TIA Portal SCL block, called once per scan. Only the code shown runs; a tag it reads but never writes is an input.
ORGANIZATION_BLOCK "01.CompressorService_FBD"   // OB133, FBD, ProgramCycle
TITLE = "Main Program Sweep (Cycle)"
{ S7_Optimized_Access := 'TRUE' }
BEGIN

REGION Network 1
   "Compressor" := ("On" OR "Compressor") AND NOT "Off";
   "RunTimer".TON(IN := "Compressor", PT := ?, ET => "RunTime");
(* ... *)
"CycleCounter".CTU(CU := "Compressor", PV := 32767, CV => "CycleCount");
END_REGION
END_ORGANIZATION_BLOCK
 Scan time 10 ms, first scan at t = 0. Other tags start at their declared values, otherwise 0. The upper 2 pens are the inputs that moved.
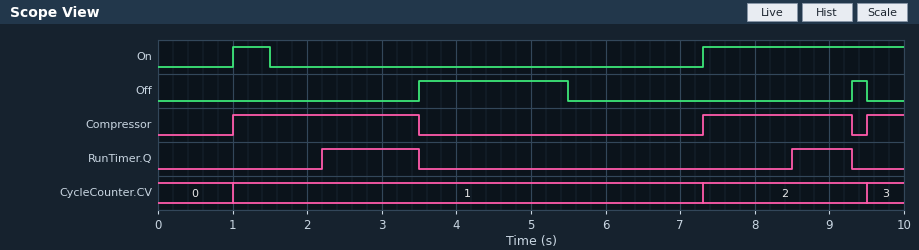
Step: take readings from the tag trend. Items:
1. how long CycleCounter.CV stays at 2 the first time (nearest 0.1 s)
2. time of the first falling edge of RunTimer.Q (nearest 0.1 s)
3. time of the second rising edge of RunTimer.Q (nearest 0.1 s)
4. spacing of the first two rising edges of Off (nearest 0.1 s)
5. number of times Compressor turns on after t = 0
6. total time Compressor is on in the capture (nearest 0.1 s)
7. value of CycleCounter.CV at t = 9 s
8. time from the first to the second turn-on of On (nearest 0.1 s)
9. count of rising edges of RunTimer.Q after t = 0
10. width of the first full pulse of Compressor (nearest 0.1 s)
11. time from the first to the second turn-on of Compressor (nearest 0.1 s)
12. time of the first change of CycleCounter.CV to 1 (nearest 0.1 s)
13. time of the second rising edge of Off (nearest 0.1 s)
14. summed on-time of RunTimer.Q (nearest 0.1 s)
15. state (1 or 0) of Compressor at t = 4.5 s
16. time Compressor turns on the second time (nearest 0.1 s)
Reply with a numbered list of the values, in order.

1. 2.2 s
2. 3.5 s
3. 8.5 s
4. 5.8 s
5. 3
6. 5.0 s
7. 2
8. 6.3 s
9. 2
10. 2.5 s
11. 6.3 s
12. 1.0 s
13. 9.3 s
14. 2.1 s
15. 0
16. 7.3 s
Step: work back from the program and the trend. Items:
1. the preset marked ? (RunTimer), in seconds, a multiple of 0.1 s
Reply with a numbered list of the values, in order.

1. 1.2 s
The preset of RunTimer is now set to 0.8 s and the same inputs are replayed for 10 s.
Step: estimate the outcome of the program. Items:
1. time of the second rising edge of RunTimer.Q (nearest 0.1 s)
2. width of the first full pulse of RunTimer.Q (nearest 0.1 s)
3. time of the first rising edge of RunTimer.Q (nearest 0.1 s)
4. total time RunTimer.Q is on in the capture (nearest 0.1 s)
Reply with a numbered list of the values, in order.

1. 8.1 s
2. 1.7 s
3. 1.8 s
4. 2.9 s
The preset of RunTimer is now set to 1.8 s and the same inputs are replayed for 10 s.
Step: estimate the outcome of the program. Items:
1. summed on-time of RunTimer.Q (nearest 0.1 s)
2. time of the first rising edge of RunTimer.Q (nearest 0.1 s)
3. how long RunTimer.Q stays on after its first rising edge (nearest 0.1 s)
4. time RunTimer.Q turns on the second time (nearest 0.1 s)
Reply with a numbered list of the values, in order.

1. 0.9 s
2. 2.8 s
3. 0.7 s
4. 9.1 s
